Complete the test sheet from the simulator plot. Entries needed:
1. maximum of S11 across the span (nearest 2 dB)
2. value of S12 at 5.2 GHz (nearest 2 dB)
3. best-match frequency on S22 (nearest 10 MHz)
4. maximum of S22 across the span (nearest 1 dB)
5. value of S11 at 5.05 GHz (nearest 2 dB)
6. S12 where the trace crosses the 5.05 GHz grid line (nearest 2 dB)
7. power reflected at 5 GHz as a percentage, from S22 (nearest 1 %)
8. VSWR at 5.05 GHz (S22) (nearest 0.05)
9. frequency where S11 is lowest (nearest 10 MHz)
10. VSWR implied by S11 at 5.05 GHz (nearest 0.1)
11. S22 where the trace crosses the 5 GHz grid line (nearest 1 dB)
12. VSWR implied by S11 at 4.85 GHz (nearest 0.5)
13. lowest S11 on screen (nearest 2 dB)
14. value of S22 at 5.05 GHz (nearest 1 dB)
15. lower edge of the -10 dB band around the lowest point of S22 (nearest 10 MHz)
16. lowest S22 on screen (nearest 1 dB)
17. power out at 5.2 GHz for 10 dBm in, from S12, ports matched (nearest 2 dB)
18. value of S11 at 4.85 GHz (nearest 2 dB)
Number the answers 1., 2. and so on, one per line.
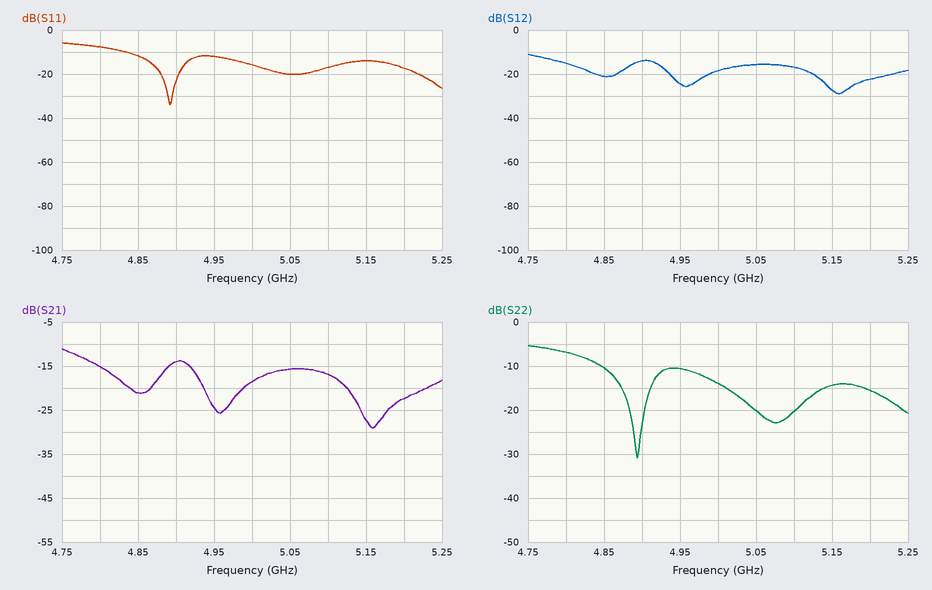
1. -6 dB
2. -22 dB
3. 4.89 GHz
4. -5 dB
5. -20 dB
6. -16 dB
7. 4 %
8. 1.20
9. 4.89 GHz
10. 1.2
11. -14 dB
12. 1.5
13. -34 dB
14. -20 dB
15. 4.85 GHz
16. -31 dB
17. -12 dBm
18. -12 dB
